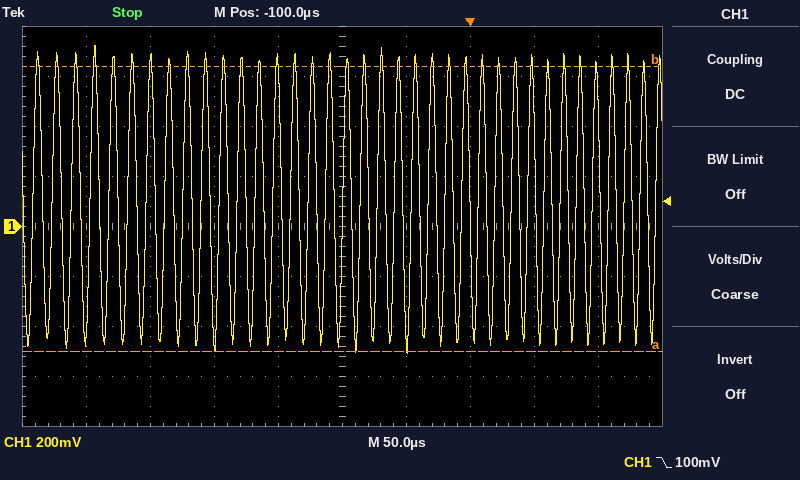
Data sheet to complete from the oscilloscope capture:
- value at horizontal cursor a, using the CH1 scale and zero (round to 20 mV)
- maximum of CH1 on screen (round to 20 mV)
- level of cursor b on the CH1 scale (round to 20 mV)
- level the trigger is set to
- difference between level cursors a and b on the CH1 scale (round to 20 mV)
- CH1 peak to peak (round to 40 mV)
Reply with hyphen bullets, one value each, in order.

- -500 mV
- 720 mV
- 640 mV
- 100 mV
- 1.14 V
- 1.24 V
